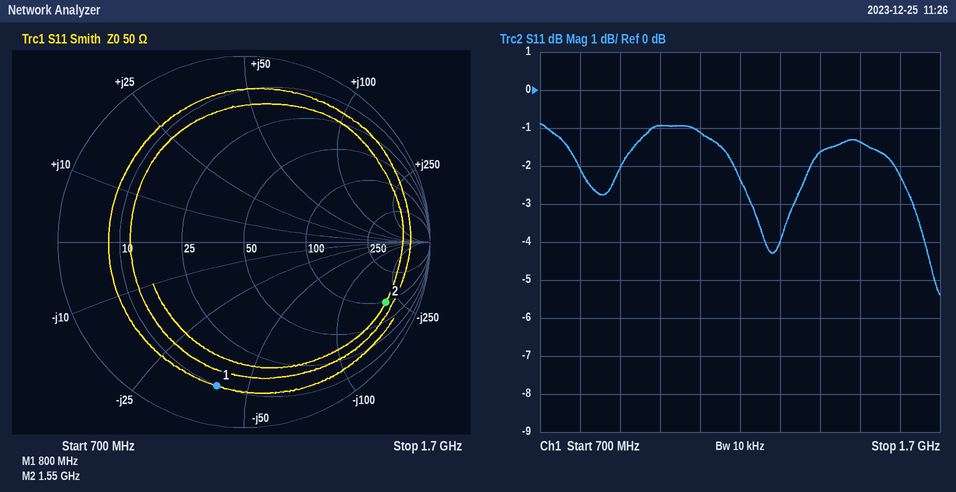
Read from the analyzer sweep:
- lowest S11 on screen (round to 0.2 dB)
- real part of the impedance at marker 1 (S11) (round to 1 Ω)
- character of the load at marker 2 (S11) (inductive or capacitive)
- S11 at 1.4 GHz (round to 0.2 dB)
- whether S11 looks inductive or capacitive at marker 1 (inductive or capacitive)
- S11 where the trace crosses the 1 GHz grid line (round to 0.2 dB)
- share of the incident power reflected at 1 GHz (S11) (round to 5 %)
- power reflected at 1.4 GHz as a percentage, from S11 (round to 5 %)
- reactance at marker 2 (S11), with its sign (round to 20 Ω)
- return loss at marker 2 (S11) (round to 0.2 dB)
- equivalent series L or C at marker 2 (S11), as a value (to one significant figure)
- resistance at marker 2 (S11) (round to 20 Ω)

-5.4 dB
10 Ω
capacitive
-1.6 dB
capacitive
-1.0 dB
80 %
70 %
-200 Ω
1.6 dB
500 fF
100 Ω
